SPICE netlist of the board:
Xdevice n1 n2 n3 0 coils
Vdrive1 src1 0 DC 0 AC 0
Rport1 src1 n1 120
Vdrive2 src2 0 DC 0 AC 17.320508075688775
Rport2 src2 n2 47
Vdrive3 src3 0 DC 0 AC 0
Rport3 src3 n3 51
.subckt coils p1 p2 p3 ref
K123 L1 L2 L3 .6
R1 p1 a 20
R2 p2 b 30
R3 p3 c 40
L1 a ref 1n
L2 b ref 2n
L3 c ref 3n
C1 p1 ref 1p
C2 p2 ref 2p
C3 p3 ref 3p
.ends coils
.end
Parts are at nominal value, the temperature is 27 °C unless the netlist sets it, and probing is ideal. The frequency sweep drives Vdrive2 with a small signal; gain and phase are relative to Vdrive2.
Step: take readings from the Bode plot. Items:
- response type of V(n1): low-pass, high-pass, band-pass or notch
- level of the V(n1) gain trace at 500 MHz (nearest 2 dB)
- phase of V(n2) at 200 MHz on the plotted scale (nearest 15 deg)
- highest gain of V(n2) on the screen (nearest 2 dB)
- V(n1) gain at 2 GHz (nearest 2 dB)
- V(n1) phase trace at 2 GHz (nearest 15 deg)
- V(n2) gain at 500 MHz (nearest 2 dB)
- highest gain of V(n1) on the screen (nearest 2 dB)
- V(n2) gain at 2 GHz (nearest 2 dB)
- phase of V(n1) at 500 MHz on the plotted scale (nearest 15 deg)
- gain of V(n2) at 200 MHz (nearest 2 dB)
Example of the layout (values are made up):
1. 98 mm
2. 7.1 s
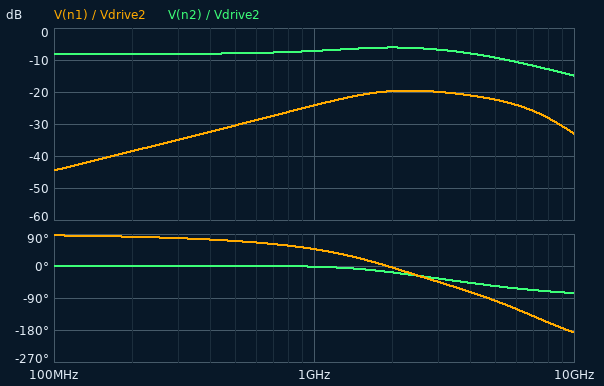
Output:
1. band-pass
2. -30 dB
3. 0 deg
4. -6 dB
5. -20 dB
6. 0 deg
7. -8 dB
8. -20 dB
9. -6 dB
10. 75 deg
11. -8 dB
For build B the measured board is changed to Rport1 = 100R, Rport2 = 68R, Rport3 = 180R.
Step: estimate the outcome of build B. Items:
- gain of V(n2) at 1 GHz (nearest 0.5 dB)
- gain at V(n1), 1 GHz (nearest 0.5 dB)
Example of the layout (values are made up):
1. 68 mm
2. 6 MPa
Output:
1. -9.0 dB
2. -26.0 dB
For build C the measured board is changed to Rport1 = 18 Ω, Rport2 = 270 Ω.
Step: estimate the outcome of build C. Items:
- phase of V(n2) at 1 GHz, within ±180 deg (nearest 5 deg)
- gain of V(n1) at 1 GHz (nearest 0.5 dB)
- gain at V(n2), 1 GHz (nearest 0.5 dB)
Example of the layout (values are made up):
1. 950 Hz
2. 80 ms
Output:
1. -5 deg
2. -41.0 dB
3. -18.5 dB
